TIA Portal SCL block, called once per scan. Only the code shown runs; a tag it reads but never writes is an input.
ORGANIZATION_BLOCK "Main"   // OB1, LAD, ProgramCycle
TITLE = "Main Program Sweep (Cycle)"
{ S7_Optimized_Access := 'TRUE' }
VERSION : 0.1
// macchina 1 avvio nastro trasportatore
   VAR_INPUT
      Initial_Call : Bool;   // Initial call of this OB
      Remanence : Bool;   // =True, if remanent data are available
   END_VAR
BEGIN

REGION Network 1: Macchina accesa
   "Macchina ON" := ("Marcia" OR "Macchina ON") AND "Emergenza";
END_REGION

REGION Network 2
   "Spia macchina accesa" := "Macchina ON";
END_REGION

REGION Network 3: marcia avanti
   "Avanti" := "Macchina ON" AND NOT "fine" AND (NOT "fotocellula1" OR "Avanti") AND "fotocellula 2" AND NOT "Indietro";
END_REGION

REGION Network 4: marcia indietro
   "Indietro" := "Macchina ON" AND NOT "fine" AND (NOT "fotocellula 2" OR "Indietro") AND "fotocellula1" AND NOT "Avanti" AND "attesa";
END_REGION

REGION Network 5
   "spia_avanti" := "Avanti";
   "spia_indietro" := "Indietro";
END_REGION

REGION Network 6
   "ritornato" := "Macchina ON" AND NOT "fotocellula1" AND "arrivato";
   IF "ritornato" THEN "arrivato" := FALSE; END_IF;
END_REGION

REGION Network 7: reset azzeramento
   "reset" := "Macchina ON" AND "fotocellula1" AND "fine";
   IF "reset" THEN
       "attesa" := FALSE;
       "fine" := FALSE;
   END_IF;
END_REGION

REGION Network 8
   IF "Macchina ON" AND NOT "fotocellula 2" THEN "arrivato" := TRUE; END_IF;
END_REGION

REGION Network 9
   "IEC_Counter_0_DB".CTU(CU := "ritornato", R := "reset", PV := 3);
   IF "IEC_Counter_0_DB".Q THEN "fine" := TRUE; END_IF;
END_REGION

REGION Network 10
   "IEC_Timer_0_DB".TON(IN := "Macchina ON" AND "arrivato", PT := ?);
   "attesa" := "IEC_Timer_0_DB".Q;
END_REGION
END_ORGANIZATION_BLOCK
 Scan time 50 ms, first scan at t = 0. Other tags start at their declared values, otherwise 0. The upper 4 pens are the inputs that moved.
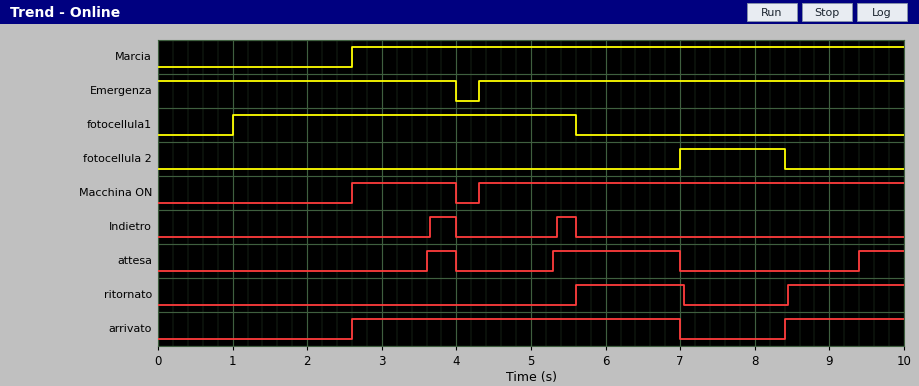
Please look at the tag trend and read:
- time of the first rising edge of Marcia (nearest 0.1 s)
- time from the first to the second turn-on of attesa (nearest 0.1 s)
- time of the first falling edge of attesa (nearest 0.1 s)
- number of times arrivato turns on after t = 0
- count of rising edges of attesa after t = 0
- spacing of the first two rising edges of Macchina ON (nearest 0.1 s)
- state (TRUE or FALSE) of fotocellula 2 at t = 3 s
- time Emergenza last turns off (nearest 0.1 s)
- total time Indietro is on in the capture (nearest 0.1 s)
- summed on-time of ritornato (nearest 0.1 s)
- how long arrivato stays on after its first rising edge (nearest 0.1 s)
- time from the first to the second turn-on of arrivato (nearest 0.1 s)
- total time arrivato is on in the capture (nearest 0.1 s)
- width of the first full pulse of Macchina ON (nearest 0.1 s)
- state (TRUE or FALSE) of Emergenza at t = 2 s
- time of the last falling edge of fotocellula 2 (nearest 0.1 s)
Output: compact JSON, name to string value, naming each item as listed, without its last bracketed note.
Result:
{"time of the first rising edge of Marcia": "2.6 s", "time from the first to the second turn-on of attesa": "1.7 s", "time of the first falling edge of attesa": "4.0 s", "number of times arrivato turns on after t = 0": "2", "count of rising edges of attesa after t = 0": "3", "spacing of the first two rising edges of Macchina ON": "1.7 s", "state (TRUE or FALSE) of fotocellula 2 at t = 3 s": "FALSE", "time Emergenza last turns off": "4.0 s", "total time Indietro is on in the capture": "0.6 s", "summed on-time of ritornato": "3.0 s", "how long arrivato stays on after its first rising edge": "4.4 s", "time from the first to the second turn-on of arrivato": "5.8 s", "total time arrivato is on in the capture": "6.0 s", "width of the first full pulse of Macchina ON": "1.4 s", "state (TRUE or FALSE) of Emergenza at t = 2 s": "TRUE", "time of the last falling edge of fotocellula 2": "8.4 s"}
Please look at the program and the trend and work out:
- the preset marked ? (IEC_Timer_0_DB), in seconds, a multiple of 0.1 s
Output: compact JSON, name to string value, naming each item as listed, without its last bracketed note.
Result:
{"the preset marked ? (IEC_Timer_0_DB), in seconds, a multiple of 0.1 s": "1.0 s"}
